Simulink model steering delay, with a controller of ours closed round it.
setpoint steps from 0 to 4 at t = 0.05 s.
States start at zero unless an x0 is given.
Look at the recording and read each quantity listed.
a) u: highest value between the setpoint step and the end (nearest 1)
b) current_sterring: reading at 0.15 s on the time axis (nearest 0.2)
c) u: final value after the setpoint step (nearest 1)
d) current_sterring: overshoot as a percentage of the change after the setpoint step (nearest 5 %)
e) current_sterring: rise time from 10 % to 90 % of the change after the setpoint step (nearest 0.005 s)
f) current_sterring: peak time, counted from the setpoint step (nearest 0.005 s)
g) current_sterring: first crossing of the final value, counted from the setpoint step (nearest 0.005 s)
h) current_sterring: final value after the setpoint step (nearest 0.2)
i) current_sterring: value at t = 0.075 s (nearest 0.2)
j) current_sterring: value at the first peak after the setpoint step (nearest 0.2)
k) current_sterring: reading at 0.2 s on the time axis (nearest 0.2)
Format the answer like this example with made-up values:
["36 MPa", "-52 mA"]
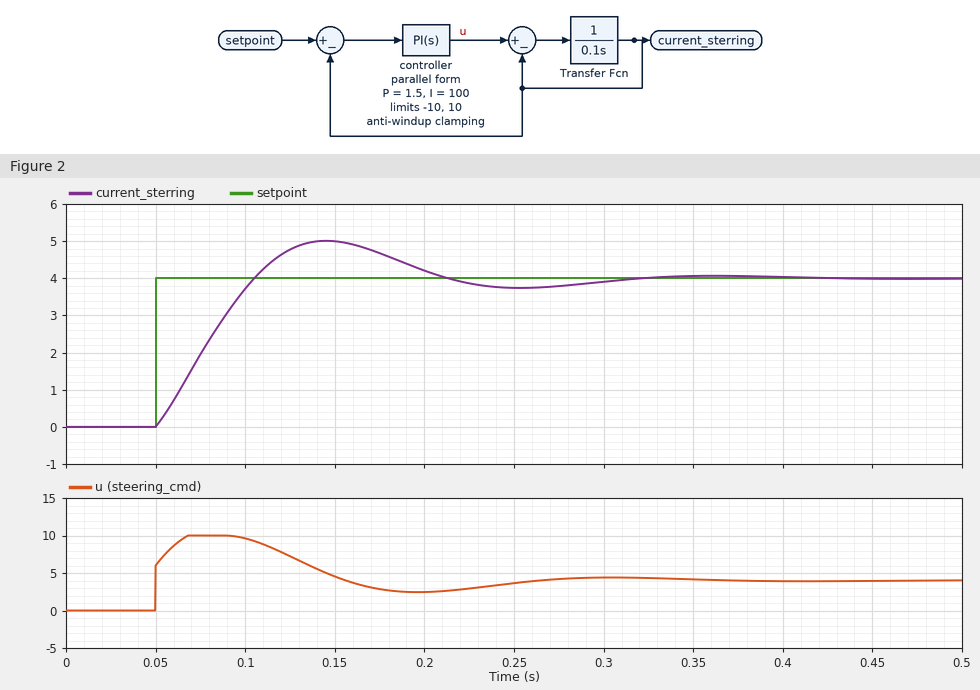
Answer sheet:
["10", "5.0", "4", "25 %", "0.040 s", "0.095 s", "0.055 s", "4.0", "2.0", "5.0", "4.2"]
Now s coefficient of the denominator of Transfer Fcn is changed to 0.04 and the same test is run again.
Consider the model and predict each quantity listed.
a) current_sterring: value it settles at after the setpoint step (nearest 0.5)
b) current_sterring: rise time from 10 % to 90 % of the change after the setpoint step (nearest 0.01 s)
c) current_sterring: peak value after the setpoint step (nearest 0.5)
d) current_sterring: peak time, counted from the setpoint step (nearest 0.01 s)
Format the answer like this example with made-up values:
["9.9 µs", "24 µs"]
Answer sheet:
["4.0", "0.03 s", "4.5", "0.06 s"]
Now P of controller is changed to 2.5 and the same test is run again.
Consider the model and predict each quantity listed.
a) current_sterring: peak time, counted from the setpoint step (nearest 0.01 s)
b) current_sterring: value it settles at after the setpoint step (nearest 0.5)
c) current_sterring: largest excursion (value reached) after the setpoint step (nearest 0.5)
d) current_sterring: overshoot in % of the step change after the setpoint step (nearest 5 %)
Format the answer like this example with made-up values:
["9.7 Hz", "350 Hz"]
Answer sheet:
["0.09 s", "4.0", "4.5", "15 %"]
